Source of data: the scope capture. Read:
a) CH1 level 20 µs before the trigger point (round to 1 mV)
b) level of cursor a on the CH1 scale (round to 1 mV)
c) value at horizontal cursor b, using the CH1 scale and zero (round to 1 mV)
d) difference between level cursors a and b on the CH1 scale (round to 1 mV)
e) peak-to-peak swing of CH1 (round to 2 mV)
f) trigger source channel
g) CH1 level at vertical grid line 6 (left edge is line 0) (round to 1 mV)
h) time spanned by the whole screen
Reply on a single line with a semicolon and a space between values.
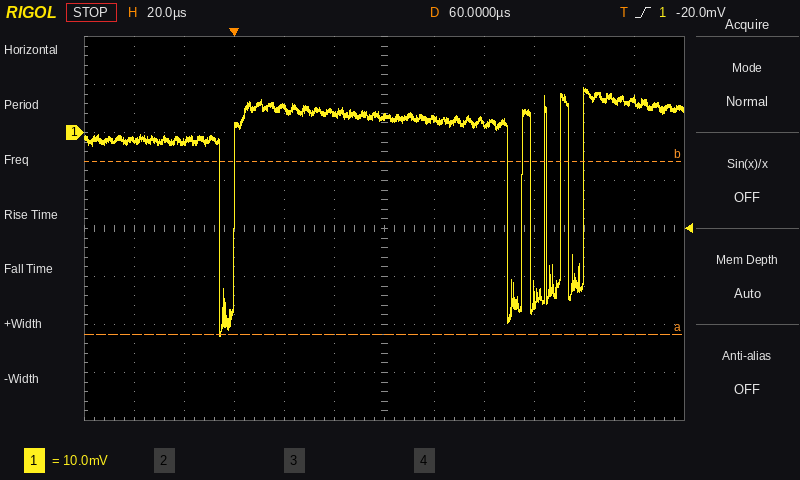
-2 mV; -42 mV; -6 mV; 36 mV; 52 mV; CH1; 3 mV; 240 µs
